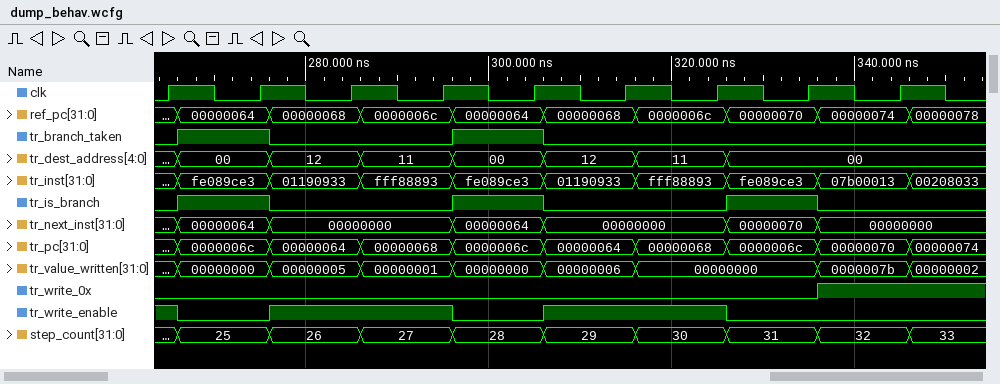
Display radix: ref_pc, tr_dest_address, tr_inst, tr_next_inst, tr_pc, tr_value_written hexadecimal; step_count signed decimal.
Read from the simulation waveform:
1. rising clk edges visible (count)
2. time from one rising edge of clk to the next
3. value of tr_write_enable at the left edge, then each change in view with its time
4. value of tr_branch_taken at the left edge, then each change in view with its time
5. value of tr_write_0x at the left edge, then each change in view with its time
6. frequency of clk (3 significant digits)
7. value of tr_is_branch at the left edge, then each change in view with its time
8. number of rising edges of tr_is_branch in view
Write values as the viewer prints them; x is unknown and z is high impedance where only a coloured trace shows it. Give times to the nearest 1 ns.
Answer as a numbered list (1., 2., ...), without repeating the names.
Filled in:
1. 9
2. 10 ns
3. 1, 0 at 266 ns, 1 at 276 ns, 0 at 296 ns, 1 at 306 ns, 0 at 326 ns
4. 0, 1 at 266 ns, 0 at 276 ns, 1 at 296 ns, 0 at 306 ns
5. 0, 1 at 336 ns
6. 100 MHz
7. 0, 1 at 266 ns, 0 at 276 ns, 1 at 296 ns, 0 at 306 ns, 1 at 326 ns, 0 at 336 ns
8. 3
